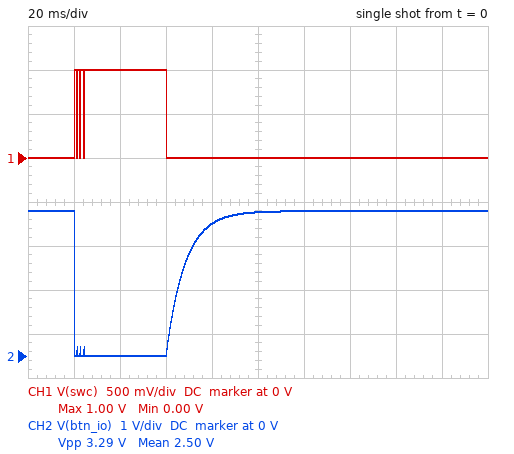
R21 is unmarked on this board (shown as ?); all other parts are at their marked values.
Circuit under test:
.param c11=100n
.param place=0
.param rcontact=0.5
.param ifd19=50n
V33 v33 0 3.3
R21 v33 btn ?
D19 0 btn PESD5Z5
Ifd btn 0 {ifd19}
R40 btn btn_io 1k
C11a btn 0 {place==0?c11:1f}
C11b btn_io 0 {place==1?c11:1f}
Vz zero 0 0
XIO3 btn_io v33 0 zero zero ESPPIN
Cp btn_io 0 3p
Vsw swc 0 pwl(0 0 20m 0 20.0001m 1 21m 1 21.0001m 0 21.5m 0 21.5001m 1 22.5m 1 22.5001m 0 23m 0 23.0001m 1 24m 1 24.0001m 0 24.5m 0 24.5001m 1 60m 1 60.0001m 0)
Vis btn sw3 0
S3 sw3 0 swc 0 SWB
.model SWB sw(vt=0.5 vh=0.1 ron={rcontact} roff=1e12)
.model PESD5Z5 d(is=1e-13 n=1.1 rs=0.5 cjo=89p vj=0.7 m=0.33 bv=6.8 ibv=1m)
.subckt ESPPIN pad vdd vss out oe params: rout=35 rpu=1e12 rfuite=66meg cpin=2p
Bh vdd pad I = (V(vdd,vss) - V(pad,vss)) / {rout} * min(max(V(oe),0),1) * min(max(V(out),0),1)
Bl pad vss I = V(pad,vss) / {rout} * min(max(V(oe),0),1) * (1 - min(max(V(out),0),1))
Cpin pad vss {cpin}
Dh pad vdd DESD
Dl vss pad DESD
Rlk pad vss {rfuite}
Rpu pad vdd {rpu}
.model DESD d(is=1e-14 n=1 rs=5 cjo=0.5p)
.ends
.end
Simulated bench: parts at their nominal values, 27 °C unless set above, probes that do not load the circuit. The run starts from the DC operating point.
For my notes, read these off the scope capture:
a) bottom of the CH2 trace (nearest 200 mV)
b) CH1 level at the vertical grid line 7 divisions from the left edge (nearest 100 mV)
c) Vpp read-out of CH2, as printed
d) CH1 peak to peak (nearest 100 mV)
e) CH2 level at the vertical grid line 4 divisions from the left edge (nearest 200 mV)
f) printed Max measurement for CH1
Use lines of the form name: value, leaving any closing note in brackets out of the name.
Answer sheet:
bottom of the CH2 trace: 0 V
CH1 level at the vertical grid line 7 divisions from the left edge: 0 V
Vpp read-out of CH2, as printed: 3.29 V
CH1 peak to peak: 1.0 V
CH2 level at the vertical grid line 4 divisions from the left edge: 3.0 V
printed Max measurement for CH1: 1.00 V
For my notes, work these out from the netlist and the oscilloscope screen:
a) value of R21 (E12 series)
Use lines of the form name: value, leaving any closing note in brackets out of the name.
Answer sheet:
value of R21: 82 kΩ
